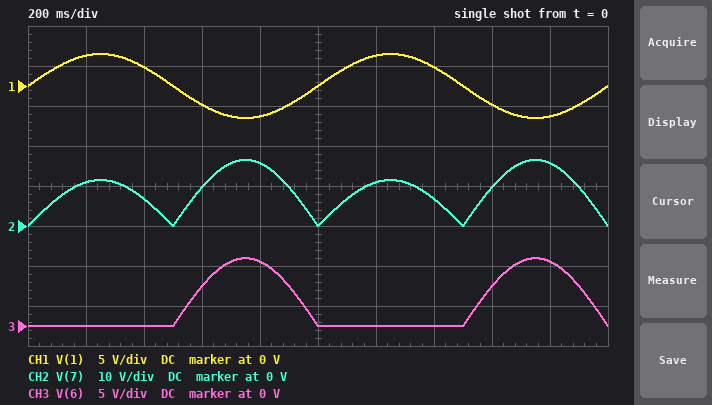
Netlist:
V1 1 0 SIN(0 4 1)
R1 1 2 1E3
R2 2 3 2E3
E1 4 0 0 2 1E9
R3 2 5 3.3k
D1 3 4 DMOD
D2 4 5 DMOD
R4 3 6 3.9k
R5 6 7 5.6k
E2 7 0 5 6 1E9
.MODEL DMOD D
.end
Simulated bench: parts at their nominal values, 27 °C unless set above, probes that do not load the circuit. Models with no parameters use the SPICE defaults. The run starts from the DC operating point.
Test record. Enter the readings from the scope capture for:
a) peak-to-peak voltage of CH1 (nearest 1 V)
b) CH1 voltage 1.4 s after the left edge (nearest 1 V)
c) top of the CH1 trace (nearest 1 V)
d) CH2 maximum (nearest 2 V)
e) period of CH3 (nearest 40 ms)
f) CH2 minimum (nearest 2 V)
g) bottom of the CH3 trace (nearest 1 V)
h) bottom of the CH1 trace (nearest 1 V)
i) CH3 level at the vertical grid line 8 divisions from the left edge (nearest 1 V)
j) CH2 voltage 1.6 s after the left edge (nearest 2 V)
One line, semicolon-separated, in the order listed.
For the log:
8 V; 2 V; 4 V; 16 V; 1.00 s; 0 V; 0 V; -4 V; 5 V; 10 V
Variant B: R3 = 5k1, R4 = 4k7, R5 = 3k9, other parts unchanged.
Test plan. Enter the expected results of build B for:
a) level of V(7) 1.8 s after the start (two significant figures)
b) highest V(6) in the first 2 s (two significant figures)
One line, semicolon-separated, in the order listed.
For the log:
17 V; 12 V
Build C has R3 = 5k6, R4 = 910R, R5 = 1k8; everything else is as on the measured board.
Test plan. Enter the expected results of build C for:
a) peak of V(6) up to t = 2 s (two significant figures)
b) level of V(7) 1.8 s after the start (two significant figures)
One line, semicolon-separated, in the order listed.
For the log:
7.7 V; 12 V
